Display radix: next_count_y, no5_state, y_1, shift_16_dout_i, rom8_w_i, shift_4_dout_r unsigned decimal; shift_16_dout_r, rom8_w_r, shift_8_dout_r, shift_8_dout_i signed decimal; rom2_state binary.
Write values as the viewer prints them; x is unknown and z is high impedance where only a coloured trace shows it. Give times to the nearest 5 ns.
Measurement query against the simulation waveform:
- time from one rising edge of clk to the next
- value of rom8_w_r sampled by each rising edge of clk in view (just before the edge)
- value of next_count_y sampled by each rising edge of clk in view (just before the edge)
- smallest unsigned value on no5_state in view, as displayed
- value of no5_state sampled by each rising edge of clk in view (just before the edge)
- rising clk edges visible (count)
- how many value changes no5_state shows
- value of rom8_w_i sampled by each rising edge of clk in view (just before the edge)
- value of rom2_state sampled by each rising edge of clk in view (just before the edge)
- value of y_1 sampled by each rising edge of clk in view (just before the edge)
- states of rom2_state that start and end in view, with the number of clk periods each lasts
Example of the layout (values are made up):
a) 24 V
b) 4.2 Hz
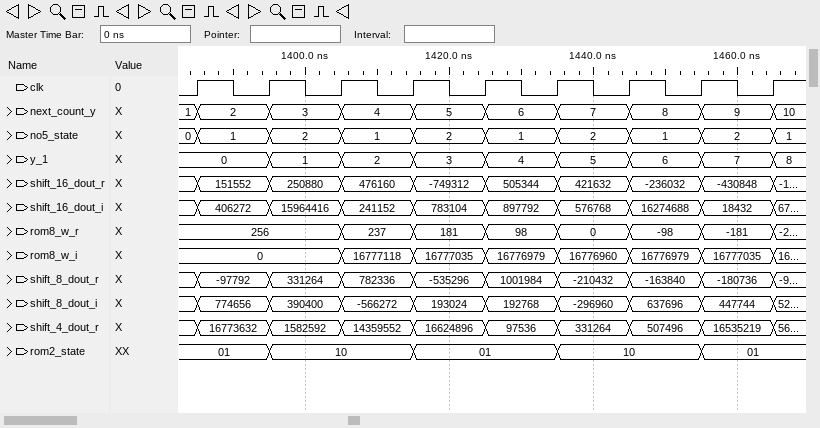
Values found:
a) 10 ns
b) 256, 256, 256, 237, 181, 98, 0, -98, -181
c) 1, 2, 3, 4, 5, 6, 7, 8, 9
d) 0
e) 0, 1, 2, 1, 2, 1, 2, 1, 2
f) 9
g) 9
h) 0, 0, 0, 16777118, 16777035, 16776979, 16776960, 16776979, 16777035
i) 01, 01, 10, 10, 01, 01, 10, 10, 01
j) 0, 0, 1, 2, 3, 4, 5, 6, 7
k) 10: 2, 01: 2, 10: 2
